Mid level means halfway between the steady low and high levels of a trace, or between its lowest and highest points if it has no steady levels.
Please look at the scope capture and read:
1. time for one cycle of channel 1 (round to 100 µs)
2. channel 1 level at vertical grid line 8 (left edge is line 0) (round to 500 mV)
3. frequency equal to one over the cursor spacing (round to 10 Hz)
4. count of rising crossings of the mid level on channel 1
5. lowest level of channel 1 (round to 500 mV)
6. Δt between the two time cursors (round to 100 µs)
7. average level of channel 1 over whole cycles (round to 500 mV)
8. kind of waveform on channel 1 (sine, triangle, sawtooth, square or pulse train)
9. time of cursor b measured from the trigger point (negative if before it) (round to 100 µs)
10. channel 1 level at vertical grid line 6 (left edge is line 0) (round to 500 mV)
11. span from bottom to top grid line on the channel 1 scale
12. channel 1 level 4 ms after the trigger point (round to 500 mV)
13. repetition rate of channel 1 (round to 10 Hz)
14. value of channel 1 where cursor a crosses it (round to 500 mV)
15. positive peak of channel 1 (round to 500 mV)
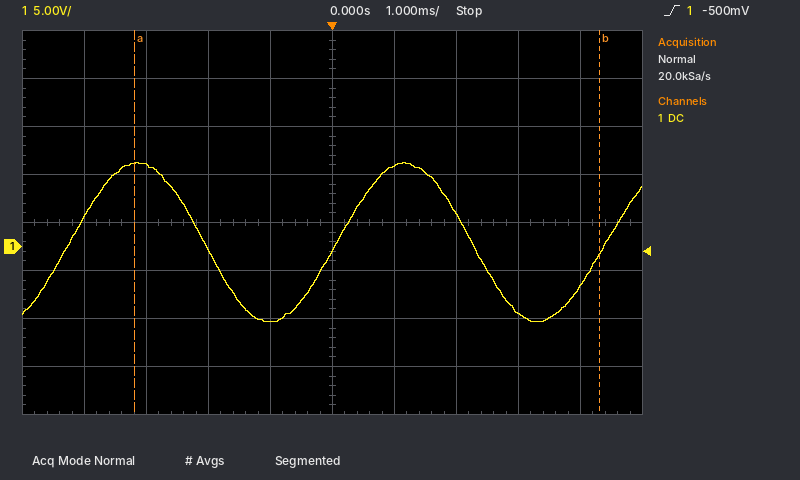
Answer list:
4.3 ms
-7.0 V
130 Hz
3
-8.0 V
7.5 ms
500 mV
sine
+4.3 ms
8.5 V
40 V
-4.0 V
230 Hz
8.5 V
9.0 V
